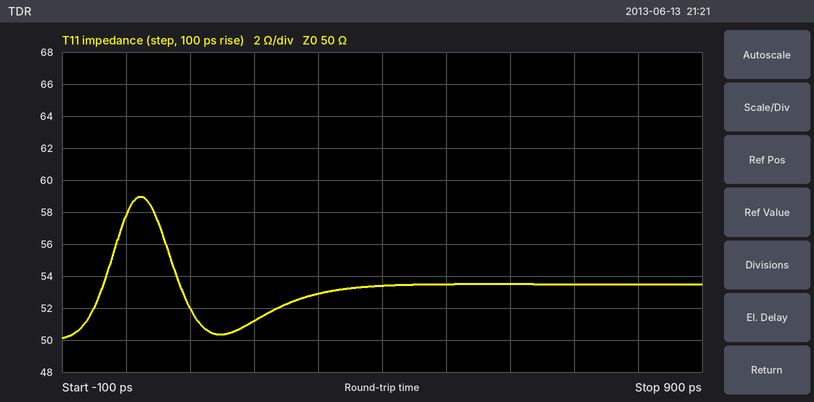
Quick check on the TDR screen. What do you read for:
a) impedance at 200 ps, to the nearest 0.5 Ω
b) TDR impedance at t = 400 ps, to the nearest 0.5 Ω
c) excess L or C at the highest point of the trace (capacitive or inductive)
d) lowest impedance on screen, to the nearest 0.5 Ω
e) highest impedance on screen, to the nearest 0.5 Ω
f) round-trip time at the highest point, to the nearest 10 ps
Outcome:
51.0 Ω
53.5 Ω
inductive
50.0 Ω
59.0 Ω
20 ps
